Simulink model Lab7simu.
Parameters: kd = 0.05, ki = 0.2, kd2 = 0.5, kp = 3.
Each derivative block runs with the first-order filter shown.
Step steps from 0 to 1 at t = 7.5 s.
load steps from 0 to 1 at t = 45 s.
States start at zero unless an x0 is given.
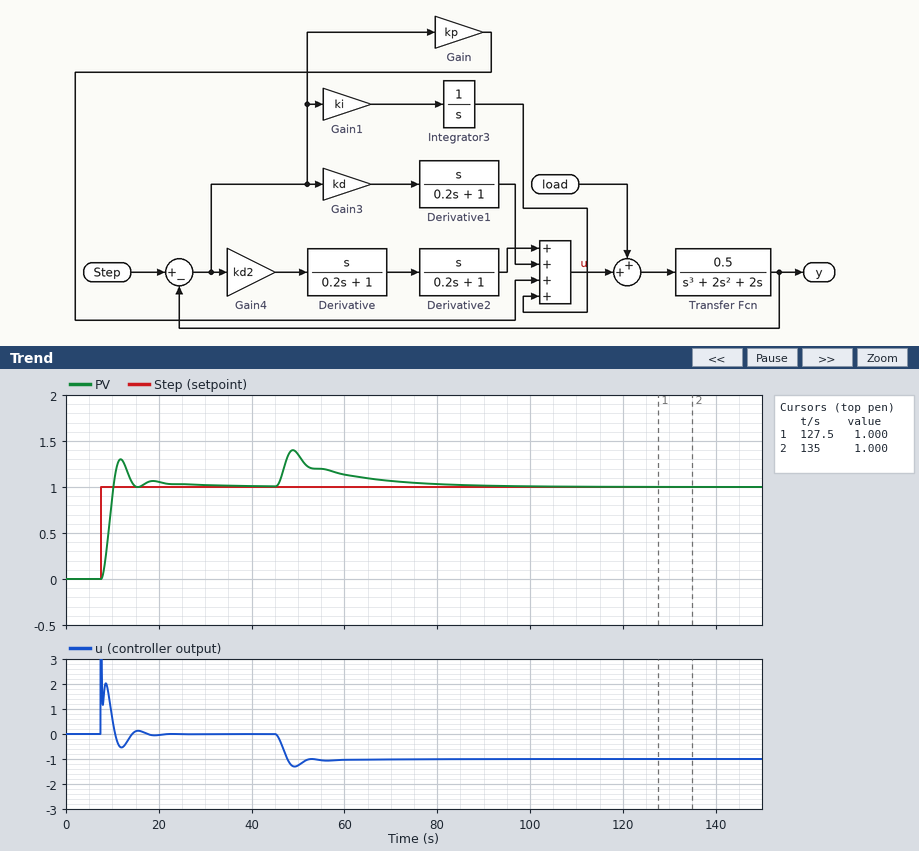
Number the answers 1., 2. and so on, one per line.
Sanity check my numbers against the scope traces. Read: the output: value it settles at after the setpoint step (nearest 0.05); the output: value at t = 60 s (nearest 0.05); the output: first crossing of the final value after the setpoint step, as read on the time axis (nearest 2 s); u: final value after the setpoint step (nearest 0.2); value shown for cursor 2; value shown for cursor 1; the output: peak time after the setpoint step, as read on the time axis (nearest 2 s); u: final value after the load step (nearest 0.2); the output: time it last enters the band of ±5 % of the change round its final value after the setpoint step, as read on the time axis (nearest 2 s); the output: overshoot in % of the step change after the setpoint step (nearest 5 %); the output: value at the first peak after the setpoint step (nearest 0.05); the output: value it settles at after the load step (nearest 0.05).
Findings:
1. 1.00
2. 1.15
3. 10 s
4. 0.0
5. 1.000
6. 1.000
7. 12 s
8. -1.0
9. 20 s
10. 30 %
11. 1.30
12. 1.00
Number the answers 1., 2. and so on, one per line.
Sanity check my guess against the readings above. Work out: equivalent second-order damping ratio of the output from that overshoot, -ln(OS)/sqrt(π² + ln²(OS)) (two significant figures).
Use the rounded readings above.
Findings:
1. 0.36
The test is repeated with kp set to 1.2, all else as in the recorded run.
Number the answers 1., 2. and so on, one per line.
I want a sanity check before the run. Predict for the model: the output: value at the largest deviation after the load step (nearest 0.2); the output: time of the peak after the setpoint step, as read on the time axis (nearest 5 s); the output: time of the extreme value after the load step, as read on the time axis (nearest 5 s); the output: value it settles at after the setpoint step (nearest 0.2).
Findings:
1. 1.6
2. 15 s
3. 50 s
4. 1.0
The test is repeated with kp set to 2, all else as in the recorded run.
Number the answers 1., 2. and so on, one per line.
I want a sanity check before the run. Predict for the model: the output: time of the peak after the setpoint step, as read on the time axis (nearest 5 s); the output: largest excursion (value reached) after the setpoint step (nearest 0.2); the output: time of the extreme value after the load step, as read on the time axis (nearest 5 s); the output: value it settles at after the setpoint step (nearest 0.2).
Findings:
1. 15 s
2. 1.2
3. 50 s
4. 1.0
